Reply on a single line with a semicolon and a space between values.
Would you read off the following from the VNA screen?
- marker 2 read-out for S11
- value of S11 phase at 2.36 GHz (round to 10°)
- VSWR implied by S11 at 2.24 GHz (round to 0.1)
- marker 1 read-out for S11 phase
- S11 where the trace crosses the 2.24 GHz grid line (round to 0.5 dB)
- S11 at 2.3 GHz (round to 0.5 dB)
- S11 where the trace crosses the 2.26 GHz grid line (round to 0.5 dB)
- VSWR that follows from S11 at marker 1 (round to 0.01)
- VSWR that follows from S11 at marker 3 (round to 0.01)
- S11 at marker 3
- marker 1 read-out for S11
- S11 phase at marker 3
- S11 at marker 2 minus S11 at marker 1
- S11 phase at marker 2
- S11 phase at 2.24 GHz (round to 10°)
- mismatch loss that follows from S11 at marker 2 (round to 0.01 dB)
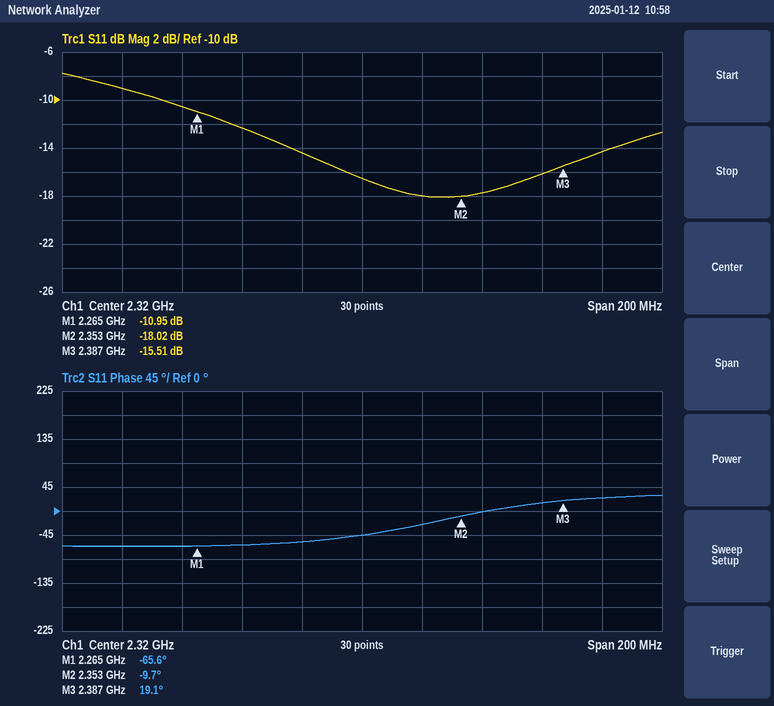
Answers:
-18.02 dB; 0°; 2.1; -65.6°; -9.0 dB; -14.5 dB; -10.5 dB; 1.79; 1.40; -15.51 dB; -10.95 dB; 19.1°; -7.07 dB; -9.7°; -70°; 0.07 dB
